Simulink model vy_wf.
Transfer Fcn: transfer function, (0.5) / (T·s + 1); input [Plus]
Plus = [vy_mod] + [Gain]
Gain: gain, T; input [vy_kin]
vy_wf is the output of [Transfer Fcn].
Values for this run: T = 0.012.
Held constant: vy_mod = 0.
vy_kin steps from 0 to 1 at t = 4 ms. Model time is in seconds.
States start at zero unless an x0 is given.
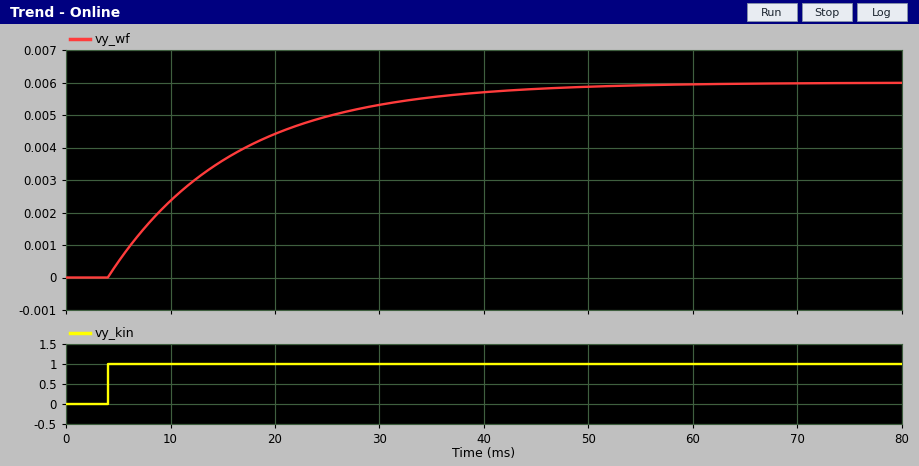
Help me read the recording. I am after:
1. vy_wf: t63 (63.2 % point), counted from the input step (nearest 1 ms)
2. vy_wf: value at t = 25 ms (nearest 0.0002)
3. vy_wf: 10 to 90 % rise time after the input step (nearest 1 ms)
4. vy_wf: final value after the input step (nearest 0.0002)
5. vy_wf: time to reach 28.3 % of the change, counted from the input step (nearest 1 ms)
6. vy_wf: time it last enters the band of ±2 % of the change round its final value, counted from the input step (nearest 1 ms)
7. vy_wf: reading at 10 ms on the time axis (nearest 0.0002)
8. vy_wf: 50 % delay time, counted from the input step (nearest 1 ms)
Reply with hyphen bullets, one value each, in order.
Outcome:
- 12 ms
- 0.0050
- 26 ms
- 0.0060
- 4 ms
- 47 ms
- 0.0024
- 8 ms
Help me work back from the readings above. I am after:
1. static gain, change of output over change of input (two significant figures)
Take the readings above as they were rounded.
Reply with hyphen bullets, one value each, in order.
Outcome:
- 0.0060
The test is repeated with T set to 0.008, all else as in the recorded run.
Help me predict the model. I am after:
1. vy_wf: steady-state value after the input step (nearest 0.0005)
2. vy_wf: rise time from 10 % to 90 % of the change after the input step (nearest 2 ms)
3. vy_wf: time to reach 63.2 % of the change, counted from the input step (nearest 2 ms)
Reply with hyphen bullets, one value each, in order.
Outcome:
- 0.0040
- 18 ms
- 8 ms
